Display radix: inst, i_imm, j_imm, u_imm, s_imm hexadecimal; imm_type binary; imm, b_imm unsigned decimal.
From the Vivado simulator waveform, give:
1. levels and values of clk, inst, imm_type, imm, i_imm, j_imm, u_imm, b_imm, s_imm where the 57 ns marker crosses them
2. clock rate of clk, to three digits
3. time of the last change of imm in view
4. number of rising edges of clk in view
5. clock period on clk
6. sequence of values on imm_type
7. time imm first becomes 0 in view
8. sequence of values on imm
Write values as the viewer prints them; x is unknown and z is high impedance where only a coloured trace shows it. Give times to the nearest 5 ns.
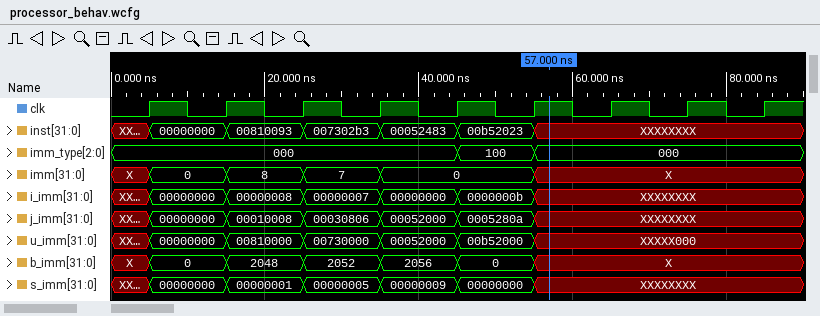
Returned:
clk=1, inst=XXXXXXXX, imm_type=000, imm=X, i_imm=XXXXXXXX, j_imm=XXXXXXXX, u_imm=XXXXX000, b_imm=X, s_imm=XXXXXXXX
100 MHz
55 ns
9
10 ns
000, 100, 000
5 ns
X, 0, 8, 7, 0, X
